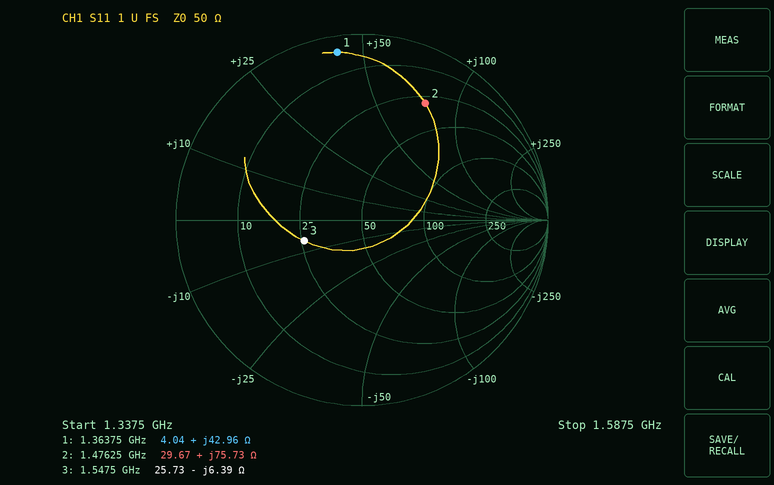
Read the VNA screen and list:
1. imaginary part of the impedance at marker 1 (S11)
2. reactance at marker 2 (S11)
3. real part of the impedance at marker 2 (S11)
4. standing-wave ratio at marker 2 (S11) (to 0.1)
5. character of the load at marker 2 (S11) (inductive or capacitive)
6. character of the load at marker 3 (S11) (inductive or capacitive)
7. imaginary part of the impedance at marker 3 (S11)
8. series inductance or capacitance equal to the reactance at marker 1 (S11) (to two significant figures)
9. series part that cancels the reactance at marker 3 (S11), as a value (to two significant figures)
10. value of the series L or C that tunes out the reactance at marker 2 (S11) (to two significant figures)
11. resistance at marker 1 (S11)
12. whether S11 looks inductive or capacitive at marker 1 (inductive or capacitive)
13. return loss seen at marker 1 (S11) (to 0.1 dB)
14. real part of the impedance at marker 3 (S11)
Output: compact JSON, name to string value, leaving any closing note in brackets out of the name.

{"imaginary part of the impedance at marker 1": "+42.96 Ω", "reactance at marker 2": "+75.73 Ω", "real part of the impedance at marker 2": "29.67 Ω", "standing-wave ratio at marker 2 (S11)": "6.0", "character of the load at marker 2 (S11)": "inductive", "character of the load at marker 3 (S11)": "capacitive", "imaginary part of the impedance at marker 3": "-6.39 Ω", "series inductance or capacitance equal to the reactance at marker 1 (S11)": "5.0 nH", "series part that cancels the reactance at marker 3 (S11), as a value": "660 pH", "value of the series L or C that tunes out the reactance at marker 2 (S11)": "1.4 pF", "resistance at marker 1": "4.04 Ω", "whether S11 looks inductive or capacitive at marker 1": "inductive", "return loss seen at marker 1 (S11)": "0.8 dB", "real part of the impedance at marker 3": "25.73 Ω"}
